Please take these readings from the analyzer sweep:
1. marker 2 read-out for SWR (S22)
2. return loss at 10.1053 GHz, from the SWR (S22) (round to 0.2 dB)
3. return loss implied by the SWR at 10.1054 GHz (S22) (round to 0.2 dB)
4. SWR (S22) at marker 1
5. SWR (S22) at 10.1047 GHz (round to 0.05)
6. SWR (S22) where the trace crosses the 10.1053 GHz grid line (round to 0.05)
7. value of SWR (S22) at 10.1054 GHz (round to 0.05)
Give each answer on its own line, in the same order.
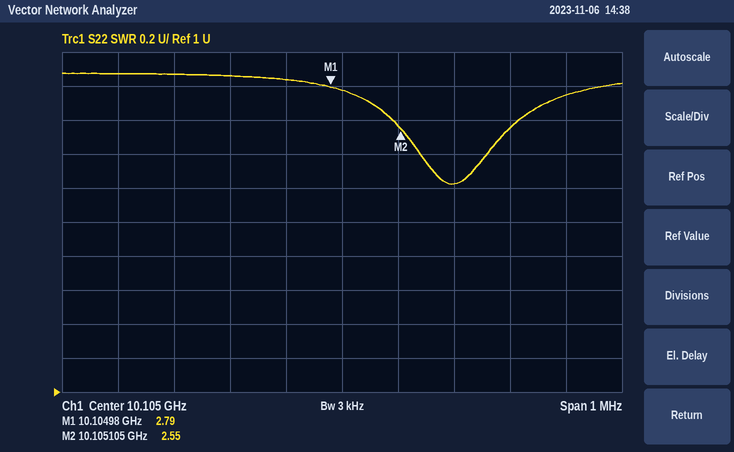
2.55
7.2 dB
6.6 dB
2.79
2.85
2.55
2.75
